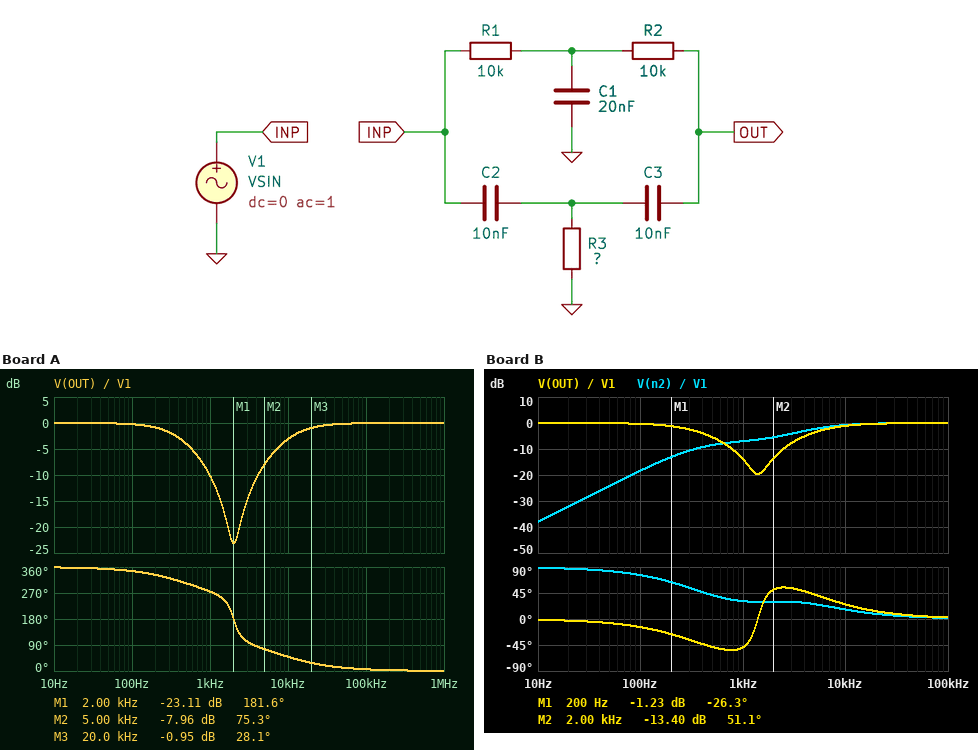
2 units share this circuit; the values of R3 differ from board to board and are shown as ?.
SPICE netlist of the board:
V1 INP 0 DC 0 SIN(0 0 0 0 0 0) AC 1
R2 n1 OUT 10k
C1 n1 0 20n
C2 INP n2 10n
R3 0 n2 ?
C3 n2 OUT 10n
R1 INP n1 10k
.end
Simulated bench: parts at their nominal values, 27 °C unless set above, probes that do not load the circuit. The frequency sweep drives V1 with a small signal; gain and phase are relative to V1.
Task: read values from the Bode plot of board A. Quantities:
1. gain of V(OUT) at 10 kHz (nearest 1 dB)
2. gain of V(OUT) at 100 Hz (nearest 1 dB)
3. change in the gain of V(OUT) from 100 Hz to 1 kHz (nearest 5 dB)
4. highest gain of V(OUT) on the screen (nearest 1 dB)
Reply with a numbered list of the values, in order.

1. -3 dB
2. 0 dB
3. -10 dB
4. 0 dB
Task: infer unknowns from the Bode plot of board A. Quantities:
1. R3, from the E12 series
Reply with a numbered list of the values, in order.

1. 2.2 kΩ
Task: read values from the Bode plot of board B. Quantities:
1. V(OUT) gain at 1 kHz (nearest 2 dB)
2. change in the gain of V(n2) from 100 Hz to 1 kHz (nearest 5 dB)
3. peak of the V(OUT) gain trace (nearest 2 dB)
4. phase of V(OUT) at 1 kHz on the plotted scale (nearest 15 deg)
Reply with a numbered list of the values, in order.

1. -14 dB
2. 10 dB
3. 0 dB
4. -45 deg
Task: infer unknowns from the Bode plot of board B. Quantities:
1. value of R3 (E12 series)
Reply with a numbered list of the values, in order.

1. 10 kΩ
